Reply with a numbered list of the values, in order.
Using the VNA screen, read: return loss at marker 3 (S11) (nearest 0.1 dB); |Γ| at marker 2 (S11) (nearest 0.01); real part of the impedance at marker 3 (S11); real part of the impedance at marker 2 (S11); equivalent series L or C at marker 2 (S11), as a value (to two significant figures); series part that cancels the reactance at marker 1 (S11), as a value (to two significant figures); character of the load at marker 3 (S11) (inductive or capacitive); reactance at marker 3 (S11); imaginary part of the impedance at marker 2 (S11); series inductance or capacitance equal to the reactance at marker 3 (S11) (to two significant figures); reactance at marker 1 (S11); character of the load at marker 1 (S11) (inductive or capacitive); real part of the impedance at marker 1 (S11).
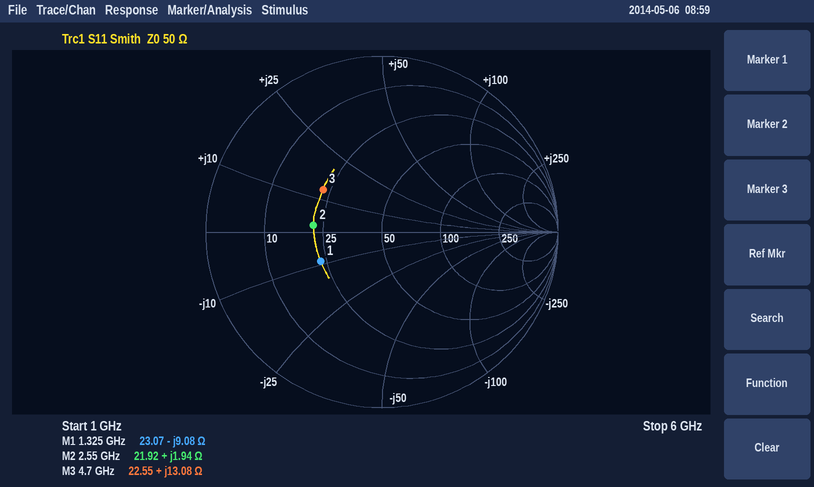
1. 7.7 dB
2. 0.39
3. 22.55 Ω
4. 21.92 Ω
5. 120 pH
6. 1.1 nH
7. inductive
8. +13.08 Ω
9. +1.94 Ω
10. 440 pH
11. -9.08 Ω
12. capacitive
13. 23.07 Ω
